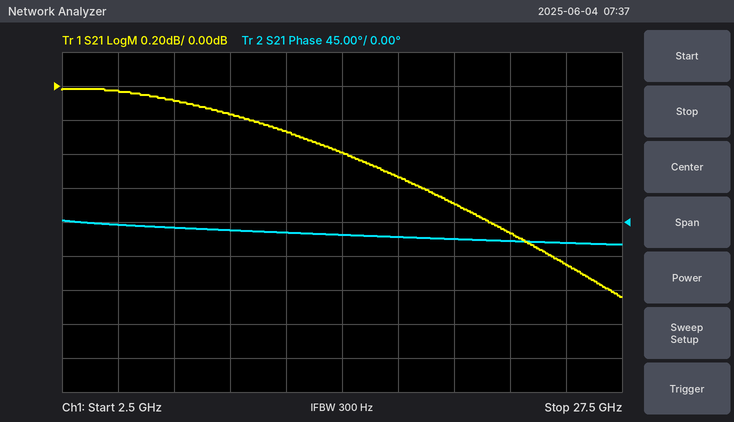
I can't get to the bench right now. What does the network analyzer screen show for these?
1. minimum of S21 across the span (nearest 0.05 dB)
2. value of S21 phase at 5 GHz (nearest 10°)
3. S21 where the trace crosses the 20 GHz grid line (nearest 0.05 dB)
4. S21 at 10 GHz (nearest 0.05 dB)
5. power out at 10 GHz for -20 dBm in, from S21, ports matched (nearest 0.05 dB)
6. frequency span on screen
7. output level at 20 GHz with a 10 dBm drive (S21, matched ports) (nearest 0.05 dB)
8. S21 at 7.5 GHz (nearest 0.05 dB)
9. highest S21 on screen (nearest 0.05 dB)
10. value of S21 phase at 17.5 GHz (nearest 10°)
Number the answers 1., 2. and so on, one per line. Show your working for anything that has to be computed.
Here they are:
1. -1.25 dB
2. 0°
3. -0.70 dB
4. -0.15 dB
5. -20 dBm + (-0.15 dB) = -20.15 dBm
6. 25 GHz
7. 10 dBm + (-0.70 dB) = 9.30 dBm
8. -0.10 dB
9. 0.00 dB
10. -20°
